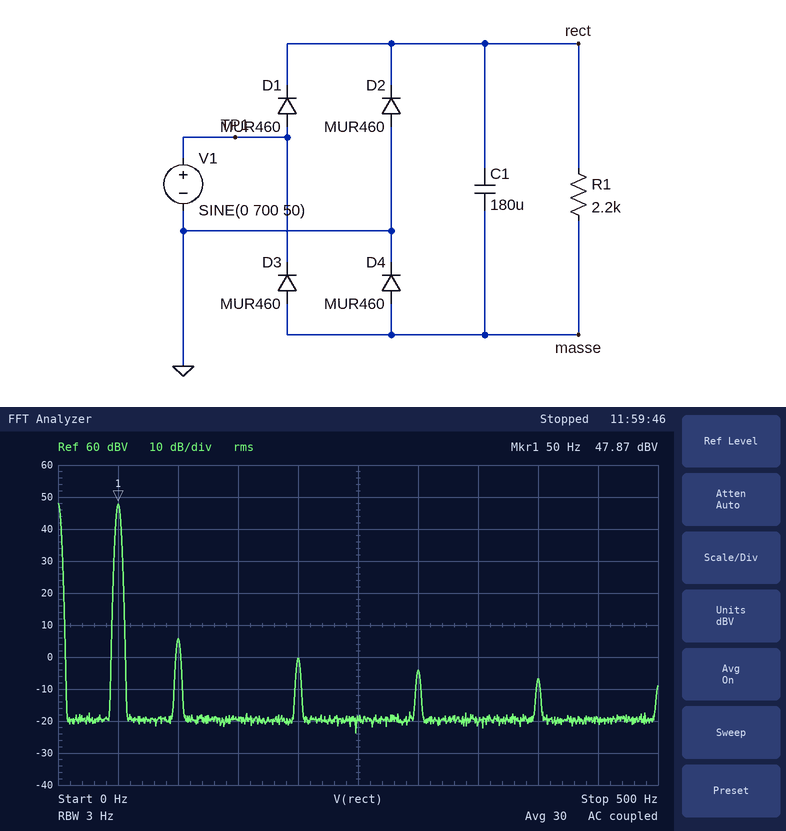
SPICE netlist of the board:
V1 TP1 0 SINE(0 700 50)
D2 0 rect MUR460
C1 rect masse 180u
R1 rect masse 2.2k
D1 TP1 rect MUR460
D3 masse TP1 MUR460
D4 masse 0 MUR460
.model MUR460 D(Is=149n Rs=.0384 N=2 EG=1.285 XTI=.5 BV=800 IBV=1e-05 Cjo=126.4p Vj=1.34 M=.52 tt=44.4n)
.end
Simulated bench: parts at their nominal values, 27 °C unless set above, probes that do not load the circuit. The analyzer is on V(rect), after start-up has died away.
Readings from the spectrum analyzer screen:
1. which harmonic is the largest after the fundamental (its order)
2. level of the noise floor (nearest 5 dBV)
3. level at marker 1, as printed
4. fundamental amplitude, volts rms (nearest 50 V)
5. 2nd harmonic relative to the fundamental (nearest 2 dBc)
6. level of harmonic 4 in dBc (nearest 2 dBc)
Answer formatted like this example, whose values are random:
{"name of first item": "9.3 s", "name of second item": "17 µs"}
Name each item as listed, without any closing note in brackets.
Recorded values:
{"which harmonic is the largest after the fundamental": "2", "level of the noise floor": "-20 dBV", "level at marker 1, as printed": "47.87 dBV", "fundamental amplitude, volts rms": "250 V", "2nd harmonic relative to the fundamental": "-42 dBc", "level of harmonic 4 in dBc": "-48 dBc"}
